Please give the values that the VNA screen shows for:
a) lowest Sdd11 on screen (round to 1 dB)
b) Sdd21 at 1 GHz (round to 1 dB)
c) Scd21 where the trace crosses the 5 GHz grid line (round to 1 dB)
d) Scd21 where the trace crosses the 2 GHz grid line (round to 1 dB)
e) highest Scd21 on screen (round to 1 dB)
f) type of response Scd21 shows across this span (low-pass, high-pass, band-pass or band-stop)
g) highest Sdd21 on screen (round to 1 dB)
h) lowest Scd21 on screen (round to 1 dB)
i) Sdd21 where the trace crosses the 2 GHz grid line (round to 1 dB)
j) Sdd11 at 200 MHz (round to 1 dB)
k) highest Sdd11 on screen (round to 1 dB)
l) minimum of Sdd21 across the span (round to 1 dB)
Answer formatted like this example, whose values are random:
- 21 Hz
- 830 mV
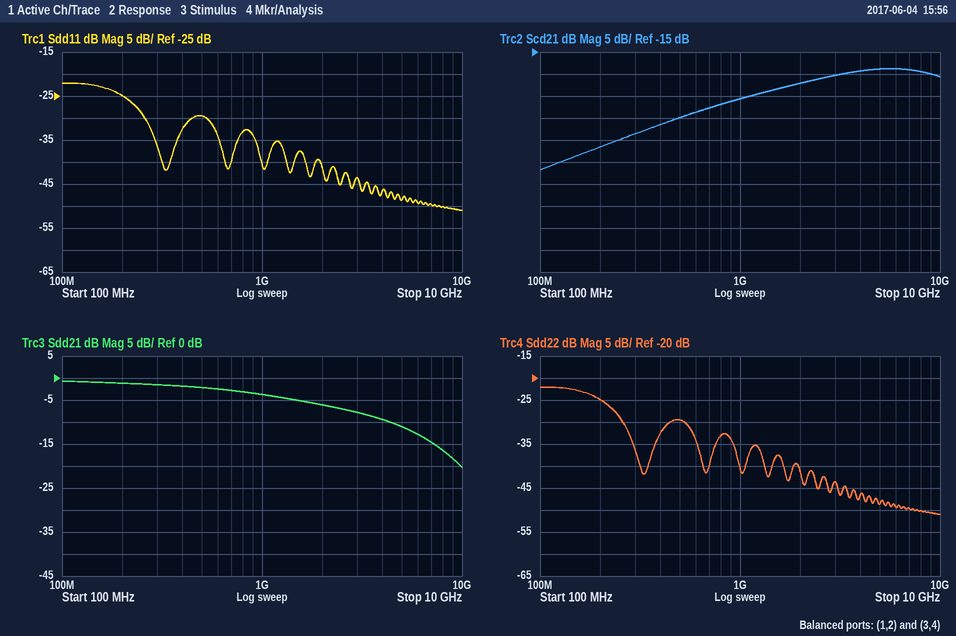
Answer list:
- -51 dB
- -4 dB
- -19 dB
- -22 dB
- -19 dB
- high-pass
- -1 dB
- -42 dB
- -6 dB
- -25 dB
- -22 dB
- -20 dB
